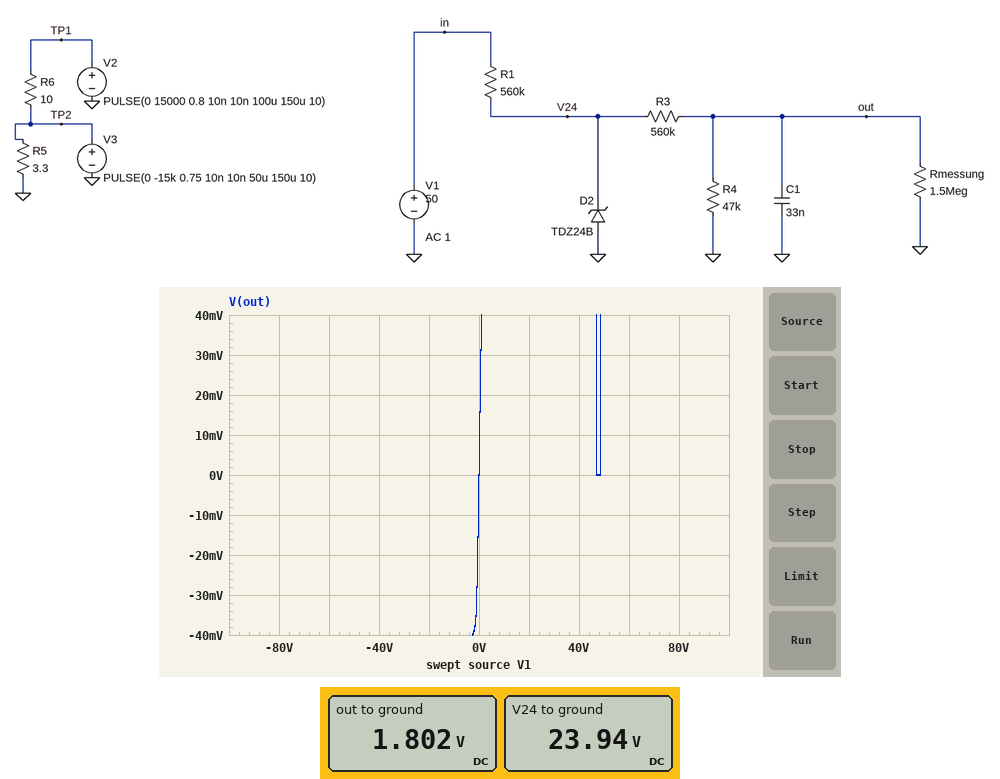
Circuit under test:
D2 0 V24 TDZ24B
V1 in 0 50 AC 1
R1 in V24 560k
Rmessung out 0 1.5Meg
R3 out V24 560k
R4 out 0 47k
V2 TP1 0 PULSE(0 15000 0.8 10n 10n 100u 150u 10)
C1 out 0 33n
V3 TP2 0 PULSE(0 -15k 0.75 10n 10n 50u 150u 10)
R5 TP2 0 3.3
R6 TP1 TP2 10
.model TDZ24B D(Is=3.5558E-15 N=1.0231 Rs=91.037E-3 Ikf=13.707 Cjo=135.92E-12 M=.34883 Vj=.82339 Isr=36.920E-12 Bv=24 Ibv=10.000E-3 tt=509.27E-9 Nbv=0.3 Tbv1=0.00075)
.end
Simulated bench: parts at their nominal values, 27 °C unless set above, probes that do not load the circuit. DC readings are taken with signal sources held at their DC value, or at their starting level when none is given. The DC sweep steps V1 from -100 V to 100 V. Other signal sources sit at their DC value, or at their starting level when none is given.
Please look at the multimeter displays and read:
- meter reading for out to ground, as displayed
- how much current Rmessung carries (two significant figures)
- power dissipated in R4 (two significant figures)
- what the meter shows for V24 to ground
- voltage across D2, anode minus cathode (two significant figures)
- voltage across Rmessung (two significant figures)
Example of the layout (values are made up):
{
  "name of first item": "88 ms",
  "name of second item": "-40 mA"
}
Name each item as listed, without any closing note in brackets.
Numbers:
{
  "meter reading for out to ground, as displayed": "1.802 V",
  "how much current Rmessung carries": "1.2 µA",
  "power dissipated in R4": "69 µW",
  "what the meter shows for V24 to ground": "23.94 V",
  "voltage across D2, anode minus cathode": "-24 V",
  "voltage across Rmessung": "1.8 V"
}
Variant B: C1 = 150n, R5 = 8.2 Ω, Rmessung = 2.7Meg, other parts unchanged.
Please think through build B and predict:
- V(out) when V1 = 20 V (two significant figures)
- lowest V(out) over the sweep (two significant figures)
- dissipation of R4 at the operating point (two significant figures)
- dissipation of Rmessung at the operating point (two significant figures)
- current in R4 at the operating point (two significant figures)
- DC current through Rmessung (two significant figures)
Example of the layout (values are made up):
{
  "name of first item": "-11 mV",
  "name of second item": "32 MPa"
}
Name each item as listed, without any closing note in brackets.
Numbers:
{
  "V(out) when V1 = 20 V": "790 mV",
  "lowest V(out) over the sweep": "-50 mV",
  "dissipation of R4 at the operating point": "71 µW",
  "dissipation of Rmessung at the operating point": "1.2 µW",
  "current in R4 at the operating point": "39 µA",
  "DC current through Rmessung": "680 nA"
}
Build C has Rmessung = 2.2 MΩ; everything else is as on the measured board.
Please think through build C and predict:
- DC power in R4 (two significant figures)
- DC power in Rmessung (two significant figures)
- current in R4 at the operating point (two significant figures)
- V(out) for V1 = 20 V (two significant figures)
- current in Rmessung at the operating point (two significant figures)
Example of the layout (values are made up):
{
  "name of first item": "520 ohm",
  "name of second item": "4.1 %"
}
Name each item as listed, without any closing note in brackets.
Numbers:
{
  "DC power in R4": "70 µW",
  "DC power in Rmessung": "1.5 µW",
  "current in R4 at the operating point": "39 µA",
  "V(out) for V1 = 20 V": "790 mV",
  "current in Rmessung at the operating point": "830 nA"
}
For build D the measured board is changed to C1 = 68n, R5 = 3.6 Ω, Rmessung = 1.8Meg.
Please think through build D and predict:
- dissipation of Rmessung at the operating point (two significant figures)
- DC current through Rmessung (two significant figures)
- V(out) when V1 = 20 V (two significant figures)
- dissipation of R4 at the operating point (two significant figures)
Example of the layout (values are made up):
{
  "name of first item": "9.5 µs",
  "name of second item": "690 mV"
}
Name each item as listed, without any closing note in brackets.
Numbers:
{
  "dissipation of Rmessung at the operating point": "1.8 µW",
  "DC current through Rmessung": "1.0 µA",
  "V(out) when V1 = 20 V": "790 mV",
  "dissipation of R4 at the operating point": "70 µW"
}
